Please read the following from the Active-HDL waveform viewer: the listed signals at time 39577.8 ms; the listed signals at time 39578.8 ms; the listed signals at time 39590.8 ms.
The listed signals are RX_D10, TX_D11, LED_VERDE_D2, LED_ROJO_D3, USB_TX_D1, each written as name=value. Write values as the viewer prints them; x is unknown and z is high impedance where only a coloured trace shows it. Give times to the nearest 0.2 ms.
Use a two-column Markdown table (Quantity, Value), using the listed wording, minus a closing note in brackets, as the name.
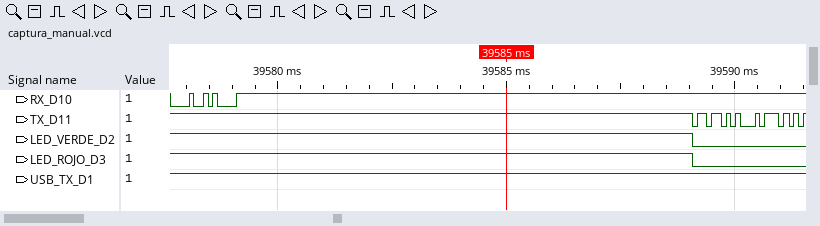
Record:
| Quantity | Value |
|---|---|
| the listed signals at time 39577.8 ms | RX_D10=0, TX_D11=1, LED_VERDE_D2=1, LED_ROJO_D3=1, USB_TX_D1=1 |
| the listed signals at time 39578.8 ms | RX_D10=0, TX_D11=1, LED_VERDE_D2=1, LED_ROJO_D3=1, USB_TX_D1=1 |
| the listed signals at time 39590.8 ms | RX_D10=1, TX_D11=1, LED_VERDE_D2=0, LED_ROJO_D3=0, USB_TX_D1=1 |
